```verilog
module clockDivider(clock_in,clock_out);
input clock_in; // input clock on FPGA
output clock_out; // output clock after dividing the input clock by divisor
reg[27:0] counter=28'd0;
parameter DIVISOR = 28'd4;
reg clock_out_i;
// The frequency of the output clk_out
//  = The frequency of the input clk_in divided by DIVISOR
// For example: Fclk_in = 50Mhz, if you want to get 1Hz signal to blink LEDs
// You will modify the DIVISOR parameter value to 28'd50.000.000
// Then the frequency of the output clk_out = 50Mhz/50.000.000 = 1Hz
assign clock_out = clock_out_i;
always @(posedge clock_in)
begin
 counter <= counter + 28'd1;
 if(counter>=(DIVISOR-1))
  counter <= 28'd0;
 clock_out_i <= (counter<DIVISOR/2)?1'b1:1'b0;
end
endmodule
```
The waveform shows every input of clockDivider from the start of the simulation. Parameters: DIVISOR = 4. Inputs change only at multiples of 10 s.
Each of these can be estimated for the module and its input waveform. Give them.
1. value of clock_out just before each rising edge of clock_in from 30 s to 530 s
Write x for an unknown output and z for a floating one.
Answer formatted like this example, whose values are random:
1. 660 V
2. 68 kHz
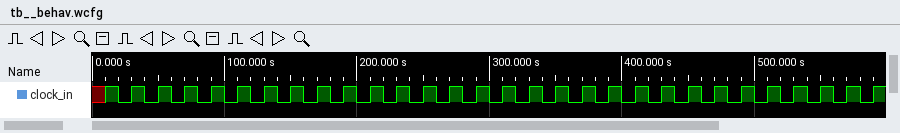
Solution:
1. 1 1 0 0 1 1 0 0 1 1 0 0 1 1 0 0 1 1 0 0 1 1 0 0 1 1
